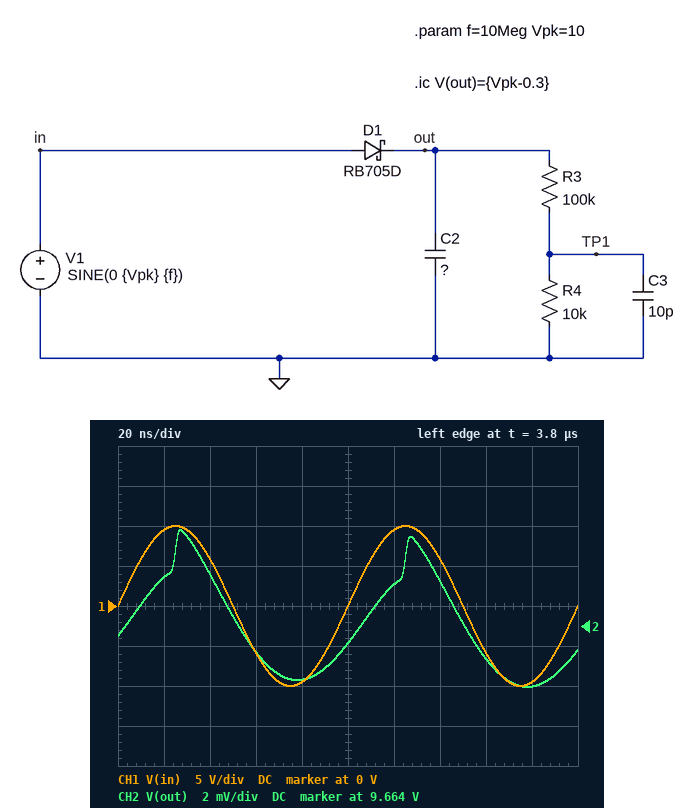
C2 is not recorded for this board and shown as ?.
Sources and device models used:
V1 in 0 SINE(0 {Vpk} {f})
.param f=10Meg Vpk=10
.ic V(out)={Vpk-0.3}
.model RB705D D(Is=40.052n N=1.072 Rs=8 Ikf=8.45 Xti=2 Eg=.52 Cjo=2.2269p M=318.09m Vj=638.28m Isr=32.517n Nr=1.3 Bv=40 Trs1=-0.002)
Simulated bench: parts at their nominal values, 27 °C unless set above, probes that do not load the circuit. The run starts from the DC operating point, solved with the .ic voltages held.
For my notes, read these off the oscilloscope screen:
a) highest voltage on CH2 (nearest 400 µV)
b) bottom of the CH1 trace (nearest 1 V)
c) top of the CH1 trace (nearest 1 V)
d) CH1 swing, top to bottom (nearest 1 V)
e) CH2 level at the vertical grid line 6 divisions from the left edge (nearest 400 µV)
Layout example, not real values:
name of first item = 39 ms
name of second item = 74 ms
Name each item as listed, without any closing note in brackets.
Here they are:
highest voltage on CH2 = 9.6688 V
bottom of the CH1 trace = -10 V
top of the CH1 trace = 10 V
CH1 swing, top to bottom = 20 V
CH2 level at the vertical grid line 6 divisions from the left edge = 9.6660 V
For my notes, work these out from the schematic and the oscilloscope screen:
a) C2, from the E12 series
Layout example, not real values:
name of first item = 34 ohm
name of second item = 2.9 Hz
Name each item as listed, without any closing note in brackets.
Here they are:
C2, from the E12 series = 3.3 nF
